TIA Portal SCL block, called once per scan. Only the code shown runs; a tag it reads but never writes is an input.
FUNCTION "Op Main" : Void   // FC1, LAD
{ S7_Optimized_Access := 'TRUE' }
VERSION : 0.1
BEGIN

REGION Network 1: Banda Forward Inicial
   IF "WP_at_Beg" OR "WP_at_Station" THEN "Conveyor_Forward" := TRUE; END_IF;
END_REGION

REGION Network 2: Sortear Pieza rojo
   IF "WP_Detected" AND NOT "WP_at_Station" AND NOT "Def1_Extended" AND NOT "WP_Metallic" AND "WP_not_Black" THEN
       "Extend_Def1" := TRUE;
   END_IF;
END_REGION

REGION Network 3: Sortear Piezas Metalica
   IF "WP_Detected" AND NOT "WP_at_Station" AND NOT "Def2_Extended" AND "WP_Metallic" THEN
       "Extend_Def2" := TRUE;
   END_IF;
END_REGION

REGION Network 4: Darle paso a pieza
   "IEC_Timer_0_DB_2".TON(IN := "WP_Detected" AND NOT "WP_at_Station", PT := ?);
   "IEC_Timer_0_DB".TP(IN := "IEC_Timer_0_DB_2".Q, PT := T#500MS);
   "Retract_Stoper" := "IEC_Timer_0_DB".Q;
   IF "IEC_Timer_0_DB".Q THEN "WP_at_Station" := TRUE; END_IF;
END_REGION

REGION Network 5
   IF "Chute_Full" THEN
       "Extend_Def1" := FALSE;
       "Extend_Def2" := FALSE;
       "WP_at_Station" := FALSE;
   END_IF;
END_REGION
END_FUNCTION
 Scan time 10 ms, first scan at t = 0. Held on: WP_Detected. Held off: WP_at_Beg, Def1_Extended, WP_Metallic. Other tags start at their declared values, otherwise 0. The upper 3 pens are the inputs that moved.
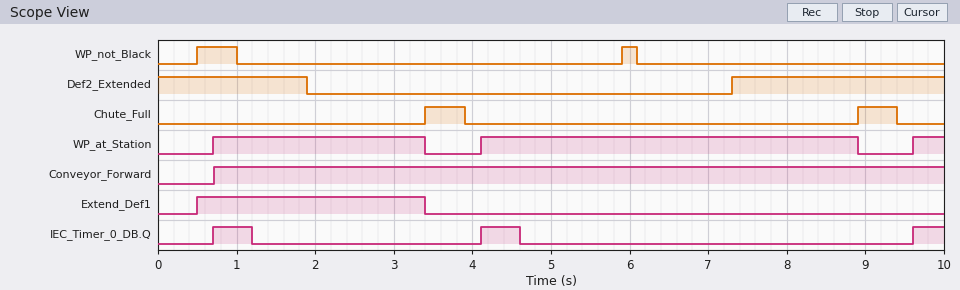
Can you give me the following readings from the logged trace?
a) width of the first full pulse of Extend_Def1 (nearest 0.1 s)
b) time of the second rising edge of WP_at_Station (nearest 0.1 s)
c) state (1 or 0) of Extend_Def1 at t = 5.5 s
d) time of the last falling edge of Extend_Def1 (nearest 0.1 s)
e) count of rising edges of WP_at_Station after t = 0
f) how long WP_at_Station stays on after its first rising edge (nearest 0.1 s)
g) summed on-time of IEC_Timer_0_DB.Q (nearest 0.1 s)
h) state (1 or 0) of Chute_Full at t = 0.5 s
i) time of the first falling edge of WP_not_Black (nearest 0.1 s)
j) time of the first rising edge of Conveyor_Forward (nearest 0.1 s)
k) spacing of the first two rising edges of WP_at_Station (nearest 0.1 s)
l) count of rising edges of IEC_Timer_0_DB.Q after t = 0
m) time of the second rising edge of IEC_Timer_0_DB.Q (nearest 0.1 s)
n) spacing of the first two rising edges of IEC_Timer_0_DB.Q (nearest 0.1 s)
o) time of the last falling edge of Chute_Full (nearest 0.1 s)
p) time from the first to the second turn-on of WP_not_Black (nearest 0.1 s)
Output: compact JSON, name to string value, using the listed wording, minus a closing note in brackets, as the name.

{"width of the first full pulse of Extend_Def1": "2.9 s", "time of the second rising edge of WP_at_Station": "4.1 s", "state (1 or 0) of Extend_Def1 at t = 5.5 s": "0", "time of the last falling edge of Extend_Def1": "3.4 s", "count of rising edges of WP_at_Station after t = 0": "3", "how long WP_at_Station stays on after its first rising edge": "2.7 s", "summed on-time of IEC_Timer_0_DB.Q": "1.4 s", "state (1 or 0) of Chute_Full at t = 0.5 s": "0", "time of the first falling edge of WP_not_Black": "1.0 s", "time of the first rising edge of Conveyor_Forward": "0.7 s", "spacing of the first two rising edges of WP_at_Station": "3.4 s", "count of rising edges of IEC_Timer_0_DB.Q after t = 0": "3", "time of the second rising edge of IEC_Timer_0_DB.Q": "4.1 s", "spacing of the first two rising edges of IEC_Timer_0_DB.Q": "3.4 s", "time of the last falling edge of Chute_Full": "9.4 s", "time from the first to the second turn-on of WP_not_Black": "5.4 s"}
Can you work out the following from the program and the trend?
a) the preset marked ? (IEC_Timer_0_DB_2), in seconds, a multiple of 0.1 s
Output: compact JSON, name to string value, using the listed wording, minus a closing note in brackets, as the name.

{"the preset marked ? (IEC_Timer_0_DB_2), in seconds, a multiple of 0.1 s": "0.7 s"}
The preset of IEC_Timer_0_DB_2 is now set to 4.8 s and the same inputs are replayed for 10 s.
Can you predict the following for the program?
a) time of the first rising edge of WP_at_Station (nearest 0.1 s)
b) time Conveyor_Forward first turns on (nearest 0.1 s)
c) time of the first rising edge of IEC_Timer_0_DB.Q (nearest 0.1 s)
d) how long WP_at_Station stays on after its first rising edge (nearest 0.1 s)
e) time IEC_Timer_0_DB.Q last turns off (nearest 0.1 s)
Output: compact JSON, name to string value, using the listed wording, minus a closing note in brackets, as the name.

{"time of the first rising edge of WP_at_Station": "4.8 s", "time Conveyor_Forward first turns on": "4.8 s", "time of the first rising edge of IEC_Timer_0_DB.Q": "4.8 s", "how long WP_at_Station stays on after its first rising edge": "4.1 s", "time IEC_Timer_0_DB.Q last turns off": "5.3 s"}
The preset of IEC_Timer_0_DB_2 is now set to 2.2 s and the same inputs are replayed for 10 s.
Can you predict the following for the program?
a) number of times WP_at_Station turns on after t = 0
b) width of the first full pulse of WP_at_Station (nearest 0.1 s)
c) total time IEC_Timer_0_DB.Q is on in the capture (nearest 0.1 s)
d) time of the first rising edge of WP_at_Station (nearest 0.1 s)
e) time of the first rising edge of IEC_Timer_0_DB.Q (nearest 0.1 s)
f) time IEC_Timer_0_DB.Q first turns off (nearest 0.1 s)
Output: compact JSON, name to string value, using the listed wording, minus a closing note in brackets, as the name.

{"number of times WP_at_Station turns on after t = 0": "2", "width of the first full pulse of WP_at_Station": "1.2 s", "total time IEC_Timer_0_DB.Q is on in the capture": "1.0 s", "time of the first rising edge of WP_at_Station": "2.2 s", "time of the first rising edge of IEC_Timer_0_DB.Q": "2.2 s", "time IEC_Timer_0_DB.Q first turns off": "2.7 s"}
